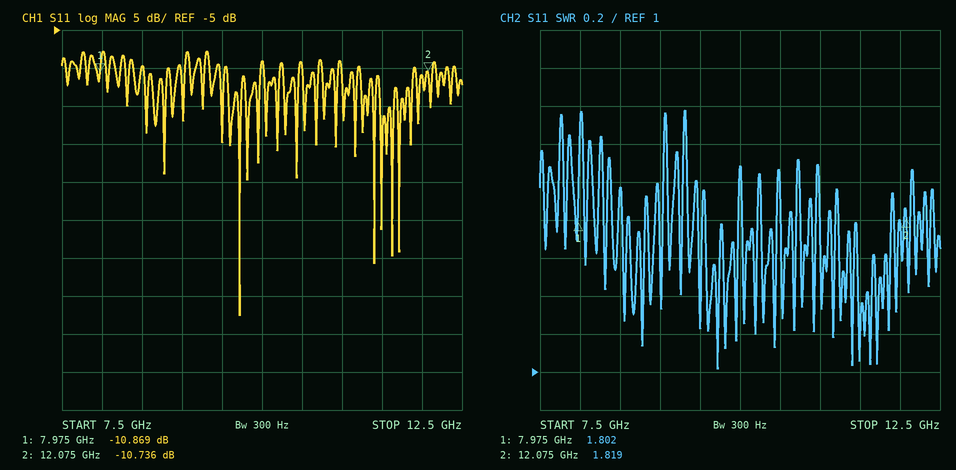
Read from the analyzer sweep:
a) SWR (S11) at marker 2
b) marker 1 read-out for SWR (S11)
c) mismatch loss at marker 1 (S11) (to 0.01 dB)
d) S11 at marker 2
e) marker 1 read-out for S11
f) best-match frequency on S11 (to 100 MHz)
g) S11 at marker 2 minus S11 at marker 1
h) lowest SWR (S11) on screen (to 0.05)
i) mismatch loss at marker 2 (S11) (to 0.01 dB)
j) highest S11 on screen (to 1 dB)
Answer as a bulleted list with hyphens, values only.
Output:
- 1.819
- 1.802
- 0.37 dB
- -10.736 dB
- -10.869 dB
- 9.7 GHz
- 0.133 dB
- 1.00
- 0.38 dB
- -8 dB
